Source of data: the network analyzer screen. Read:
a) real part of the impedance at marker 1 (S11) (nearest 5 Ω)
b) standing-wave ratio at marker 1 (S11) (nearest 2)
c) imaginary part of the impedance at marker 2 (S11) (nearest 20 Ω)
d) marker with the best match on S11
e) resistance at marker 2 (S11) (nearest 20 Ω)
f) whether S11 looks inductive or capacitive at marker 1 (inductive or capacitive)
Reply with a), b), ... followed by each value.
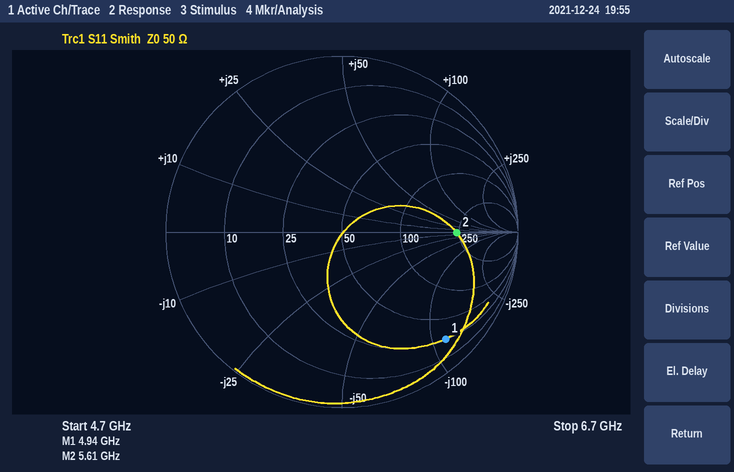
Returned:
a) 25 Ω
b) 12
c) 0 Ω
d) marker 2
e) 240 Ω
f) capacitive
